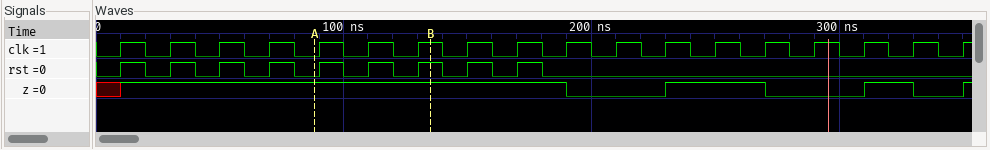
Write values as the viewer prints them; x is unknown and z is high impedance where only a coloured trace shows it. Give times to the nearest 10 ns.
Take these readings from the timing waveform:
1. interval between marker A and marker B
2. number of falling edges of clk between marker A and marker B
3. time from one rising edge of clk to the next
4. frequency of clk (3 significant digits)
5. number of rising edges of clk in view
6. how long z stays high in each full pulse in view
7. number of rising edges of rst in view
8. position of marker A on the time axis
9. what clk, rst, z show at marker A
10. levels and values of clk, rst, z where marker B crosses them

50 ns
2
20 ns
50.0 MHz
18
40 ns, 20 ns
9
90 ns
clk=0, rst=0, z=1
clk=1, rst=1, z=1
